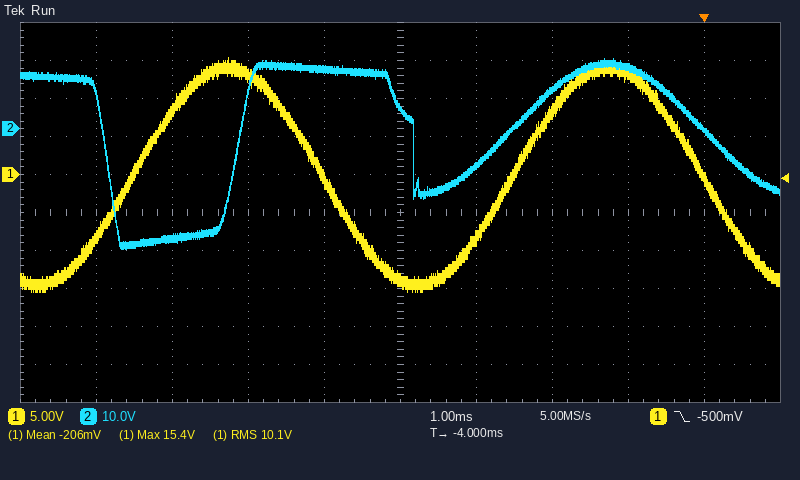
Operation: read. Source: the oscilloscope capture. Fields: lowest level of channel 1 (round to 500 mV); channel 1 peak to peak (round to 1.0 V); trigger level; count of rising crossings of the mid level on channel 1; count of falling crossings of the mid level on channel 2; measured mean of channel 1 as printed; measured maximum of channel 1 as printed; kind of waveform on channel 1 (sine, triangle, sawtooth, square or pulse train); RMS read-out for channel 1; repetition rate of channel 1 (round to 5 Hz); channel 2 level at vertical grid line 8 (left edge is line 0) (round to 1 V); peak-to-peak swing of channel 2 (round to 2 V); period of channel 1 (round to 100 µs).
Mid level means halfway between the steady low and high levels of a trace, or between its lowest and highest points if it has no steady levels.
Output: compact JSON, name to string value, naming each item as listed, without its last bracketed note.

{"lowest level of channel 1": "-15.5 V", "channel 1 peak to peak": "31.0 V", "trigger level": "-500 mV", "count of rising crossings of the mid level on channel 1": "2", "count of falling crossings of the mid level on channel 2": "3", "measured mean of channel 1 as printed": "-206 mV", "measured maximum of channel 1 as printed": "15.4 V", "kind of waveform on channel 1": "sine", "RMS read-out for channel 1": "10.1 V", "repetition rate of channel 1": "200 Hz", "channel 2 level at vertical grid line 8 (left edge is line 0)": "16 V", "peak-to-peak swing of channel 2": "50 V", "period of channel 1": "5.0 ms"}
